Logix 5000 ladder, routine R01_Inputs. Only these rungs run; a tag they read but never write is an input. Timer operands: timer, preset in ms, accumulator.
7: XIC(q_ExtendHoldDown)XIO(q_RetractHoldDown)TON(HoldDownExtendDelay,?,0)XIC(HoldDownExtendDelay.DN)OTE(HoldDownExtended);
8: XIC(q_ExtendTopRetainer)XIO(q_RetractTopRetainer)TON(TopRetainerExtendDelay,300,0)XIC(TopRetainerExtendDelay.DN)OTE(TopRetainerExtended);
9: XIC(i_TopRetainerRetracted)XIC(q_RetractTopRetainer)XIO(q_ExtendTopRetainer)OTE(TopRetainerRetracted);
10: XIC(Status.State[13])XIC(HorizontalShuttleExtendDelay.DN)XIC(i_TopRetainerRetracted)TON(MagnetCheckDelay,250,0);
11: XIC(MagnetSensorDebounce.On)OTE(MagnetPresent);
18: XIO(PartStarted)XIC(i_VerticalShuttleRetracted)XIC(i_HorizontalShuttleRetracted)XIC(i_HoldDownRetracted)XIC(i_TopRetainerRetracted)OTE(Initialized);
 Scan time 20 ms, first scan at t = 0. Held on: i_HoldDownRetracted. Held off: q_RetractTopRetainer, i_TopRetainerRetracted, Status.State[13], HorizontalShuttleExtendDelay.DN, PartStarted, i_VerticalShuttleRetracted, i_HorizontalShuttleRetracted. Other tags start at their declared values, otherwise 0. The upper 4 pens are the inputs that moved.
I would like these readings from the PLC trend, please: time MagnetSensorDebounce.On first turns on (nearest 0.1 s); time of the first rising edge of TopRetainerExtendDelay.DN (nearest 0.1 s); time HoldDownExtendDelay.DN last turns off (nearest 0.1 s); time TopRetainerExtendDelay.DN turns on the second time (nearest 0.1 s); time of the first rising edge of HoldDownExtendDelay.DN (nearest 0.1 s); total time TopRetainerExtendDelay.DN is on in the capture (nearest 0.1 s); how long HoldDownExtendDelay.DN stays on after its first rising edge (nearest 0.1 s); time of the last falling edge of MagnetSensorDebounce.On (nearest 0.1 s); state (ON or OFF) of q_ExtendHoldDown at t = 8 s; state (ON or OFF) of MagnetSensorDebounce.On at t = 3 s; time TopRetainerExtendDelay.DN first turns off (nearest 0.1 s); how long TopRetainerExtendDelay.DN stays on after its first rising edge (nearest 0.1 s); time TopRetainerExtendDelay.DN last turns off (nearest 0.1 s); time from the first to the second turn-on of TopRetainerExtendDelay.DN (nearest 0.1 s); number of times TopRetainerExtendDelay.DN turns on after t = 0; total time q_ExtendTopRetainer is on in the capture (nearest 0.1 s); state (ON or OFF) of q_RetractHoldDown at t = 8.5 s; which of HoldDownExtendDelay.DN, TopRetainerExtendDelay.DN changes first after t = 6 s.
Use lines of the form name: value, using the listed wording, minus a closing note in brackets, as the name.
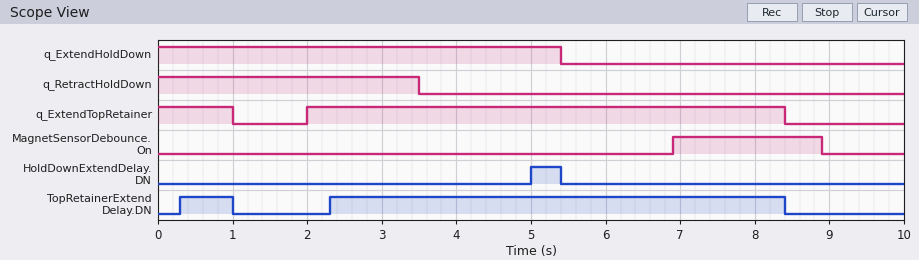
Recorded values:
time MagnetSensorDebounce.On first turns on: 6.9 s
time of the first rising edge of TopRetainerExtendDelay.DN: 0.3 s
time HoldDownExtendDelay.DN last turns off: 5.4 s
time TopRetainerExtendDelay.DN turns on the second time: 2.3 s
time of the first rising edge of HoldDownExtendDelay.DN: 5.0 s
total time TopRetainerExtendDelay.DN is on in the capture: 6.8 s
how long HoldDownExtendDelay.DN stays on after its first rising edge: 0.4 s
time of the last falling edge of MagnetSensorDebounce.On: 8.9 s
state (ON or OFF) of q_ExtendHoldDown at t = 8 s: OFF
state (ON or OFF) of MagnetSensorDebounce.On at t = 3 s: OFF
time TopRetainerExtendDelay.DN first turns off: 1.0 s
how long TopRetainerExtendDelay.DN stays on after its first rising edge: 0.7 s
time TopRetainerExtendDelay.DN last turns off: 8.4 s
time from the first to the second turn-on of TopRetainerExtendDelay.DN: 2.0 s
number of times TopRetainerExtendDelay.DN turns on after t = 0: 2
total time q_ExtendTopRetainer is on in the capture: 7.4 s
state (ON or OFF) of q_RetractHoldDown at t = 8.5 s: OFF
which of HoldDownExtendDelay.DN, TopRetainerExtendDelay.DN changes first after t = 6 s: TopRetainerExtendDelay.DN
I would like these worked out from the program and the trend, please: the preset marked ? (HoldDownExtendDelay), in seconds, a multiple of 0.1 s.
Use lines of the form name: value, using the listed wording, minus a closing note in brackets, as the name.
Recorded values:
the preset marked ? (HoldDownExtendDelay), in seconds, a multiple of 0.1 s: 1.5 s
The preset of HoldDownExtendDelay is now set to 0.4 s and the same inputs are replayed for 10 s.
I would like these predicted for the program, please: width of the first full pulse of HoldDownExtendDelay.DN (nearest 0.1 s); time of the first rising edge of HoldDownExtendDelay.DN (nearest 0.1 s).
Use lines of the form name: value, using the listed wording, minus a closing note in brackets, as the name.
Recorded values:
width of the first full pulse of HoldDownExtendDelay.DN: 1.5 s
time of the first rising edge of HoldDownExtendDelay.DN: 3.9 s
